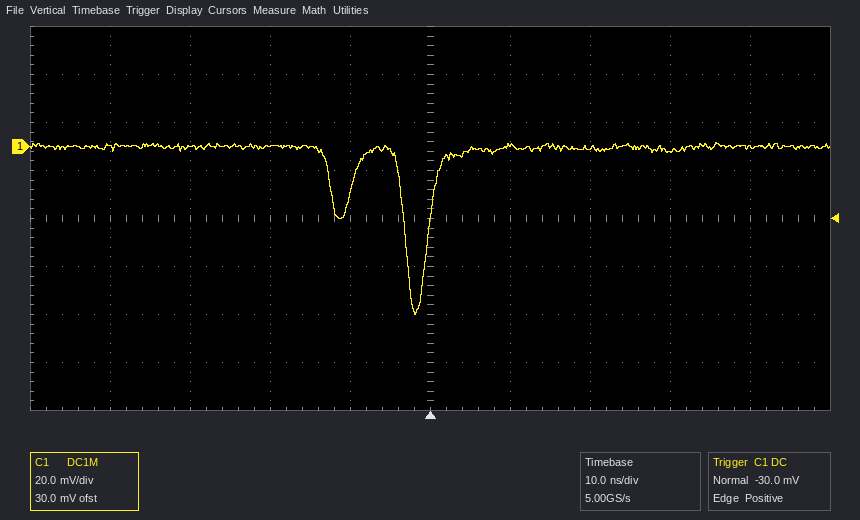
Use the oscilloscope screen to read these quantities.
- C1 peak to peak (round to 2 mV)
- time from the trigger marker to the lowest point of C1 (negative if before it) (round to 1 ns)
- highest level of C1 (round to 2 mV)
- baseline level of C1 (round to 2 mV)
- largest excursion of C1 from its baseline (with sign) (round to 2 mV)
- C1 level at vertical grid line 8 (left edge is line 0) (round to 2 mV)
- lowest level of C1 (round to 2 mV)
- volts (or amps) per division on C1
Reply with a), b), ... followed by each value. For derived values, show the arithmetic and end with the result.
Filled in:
a) 2 mV − (-70 mV) = 72 mV
b) -2 ns
c) 2 mV
d) 0 mV
e) -70 mV − (0 mV) = -70 mV
f) -2 mV
g) -70 mV
h) 20 mV
